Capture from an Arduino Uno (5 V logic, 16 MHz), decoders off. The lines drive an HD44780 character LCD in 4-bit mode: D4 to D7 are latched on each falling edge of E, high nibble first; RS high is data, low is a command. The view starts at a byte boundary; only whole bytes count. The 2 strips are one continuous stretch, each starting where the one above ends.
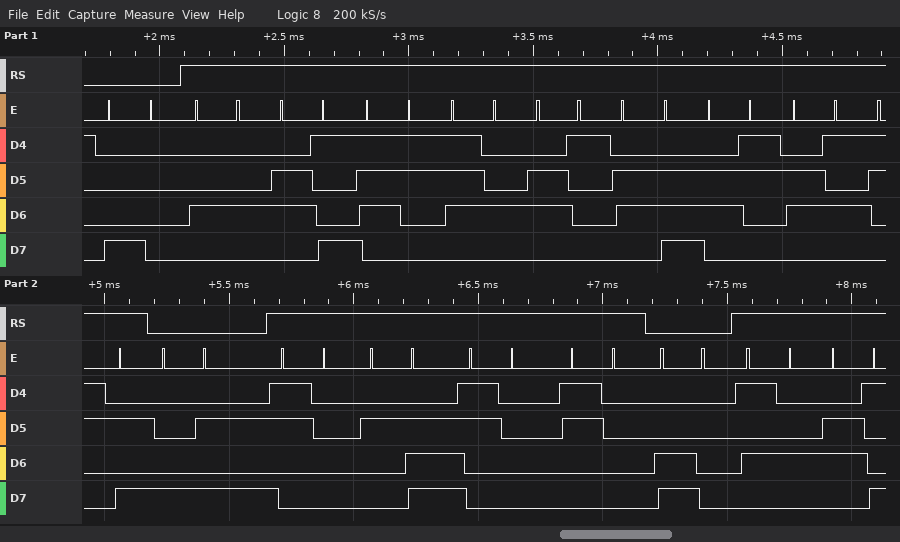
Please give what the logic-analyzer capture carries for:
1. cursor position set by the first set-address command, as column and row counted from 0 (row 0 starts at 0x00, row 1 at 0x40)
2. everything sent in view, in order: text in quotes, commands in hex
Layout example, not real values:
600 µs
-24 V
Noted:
column 0, row 0
0x80 "Distance:" 0x8A "0.00" 0xC0 "Ti"
